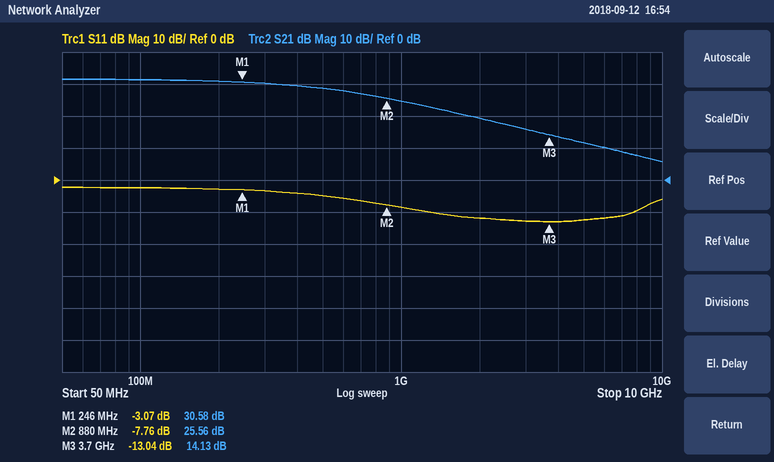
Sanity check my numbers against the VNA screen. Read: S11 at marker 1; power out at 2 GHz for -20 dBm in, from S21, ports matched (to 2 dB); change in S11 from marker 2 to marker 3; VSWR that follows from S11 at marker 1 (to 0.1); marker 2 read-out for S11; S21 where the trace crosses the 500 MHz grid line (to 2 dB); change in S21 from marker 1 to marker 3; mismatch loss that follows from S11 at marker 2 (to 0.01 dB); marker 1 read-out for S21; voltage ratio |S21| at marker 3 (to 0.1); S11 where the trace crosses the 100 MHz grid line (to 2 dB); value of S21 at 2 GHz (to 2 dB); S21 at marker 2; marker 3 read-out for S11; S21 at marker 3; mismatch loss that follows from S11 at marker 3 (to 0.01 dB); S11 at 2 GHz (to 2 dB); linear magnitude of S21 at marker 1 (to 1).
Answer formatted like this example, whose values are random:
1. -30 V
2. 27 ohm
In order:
1. -3.07 dB
2. 0 dBm
3. -5.28 dB
4. 5.7
5. -7.76 dB
6. 28 dB
7. -16.45 dB
8. 0.80 dB
9. 30.58 dB
10. 5.1
11. -2 dB
12. 20 dB
13. 25.56 dB
14. -13.04 dB
15. 14.13 dB
16. 0.22 dB
17. -12 dB
18. 34
